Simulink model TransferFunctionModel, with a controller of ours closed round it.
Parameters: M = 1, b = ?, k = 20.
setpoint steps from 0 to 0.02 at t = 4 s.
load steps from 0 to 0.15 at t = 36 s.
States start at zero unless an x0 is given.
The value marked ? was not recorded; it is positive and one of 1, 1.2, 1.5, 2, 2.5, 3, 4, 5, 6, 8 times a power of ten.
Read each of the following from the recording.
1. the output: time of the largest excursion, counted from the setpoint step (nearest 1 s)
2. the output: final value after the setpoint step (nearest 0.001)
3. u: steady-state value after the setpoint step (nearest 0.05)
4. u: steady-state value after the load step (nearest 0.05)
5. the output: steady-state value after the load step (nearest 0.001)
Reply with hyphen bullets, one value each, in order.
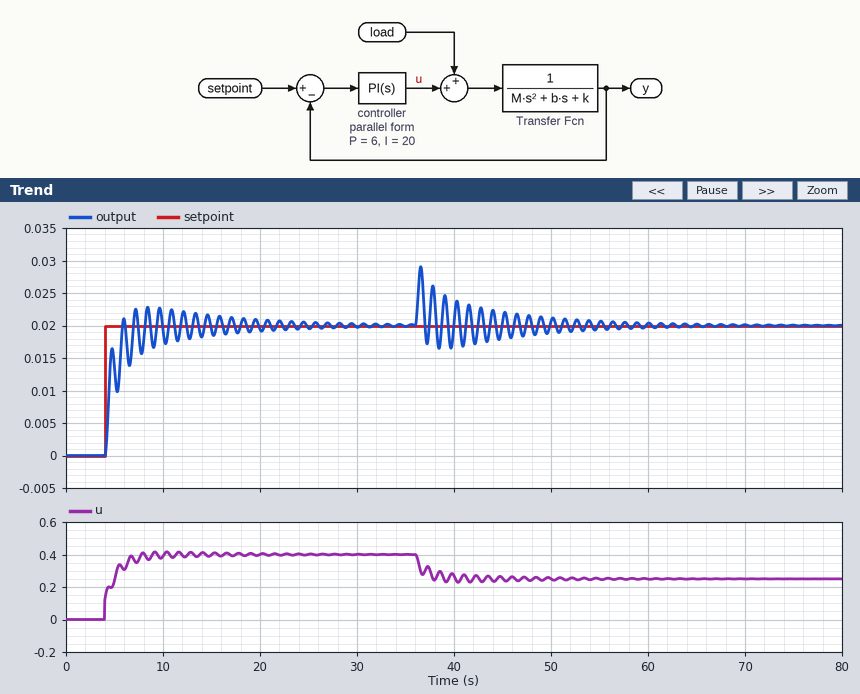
- 4 s
- 0.020
- 0.40
- 0.25
- 0.020
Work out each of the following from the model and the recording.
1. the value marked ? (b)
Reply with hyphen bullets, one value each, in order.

- 1
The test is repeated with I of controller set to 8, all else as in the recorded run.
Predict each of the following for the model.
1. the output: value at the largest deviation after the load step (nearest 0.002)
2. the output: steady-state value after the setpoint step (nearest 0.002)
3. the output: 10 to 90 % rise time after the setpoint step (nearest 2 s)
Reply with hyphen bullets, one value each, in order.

- 0.030
- 0.020
- 6 s
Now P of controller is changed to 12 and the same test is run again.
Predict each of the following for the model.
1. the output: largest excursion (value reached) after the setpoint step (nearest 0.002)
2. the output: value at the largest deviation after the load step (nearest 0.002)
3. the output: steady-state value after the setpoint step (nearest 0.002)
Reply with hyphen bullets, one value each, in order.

- 0.022
- 0.028
- 0.020
